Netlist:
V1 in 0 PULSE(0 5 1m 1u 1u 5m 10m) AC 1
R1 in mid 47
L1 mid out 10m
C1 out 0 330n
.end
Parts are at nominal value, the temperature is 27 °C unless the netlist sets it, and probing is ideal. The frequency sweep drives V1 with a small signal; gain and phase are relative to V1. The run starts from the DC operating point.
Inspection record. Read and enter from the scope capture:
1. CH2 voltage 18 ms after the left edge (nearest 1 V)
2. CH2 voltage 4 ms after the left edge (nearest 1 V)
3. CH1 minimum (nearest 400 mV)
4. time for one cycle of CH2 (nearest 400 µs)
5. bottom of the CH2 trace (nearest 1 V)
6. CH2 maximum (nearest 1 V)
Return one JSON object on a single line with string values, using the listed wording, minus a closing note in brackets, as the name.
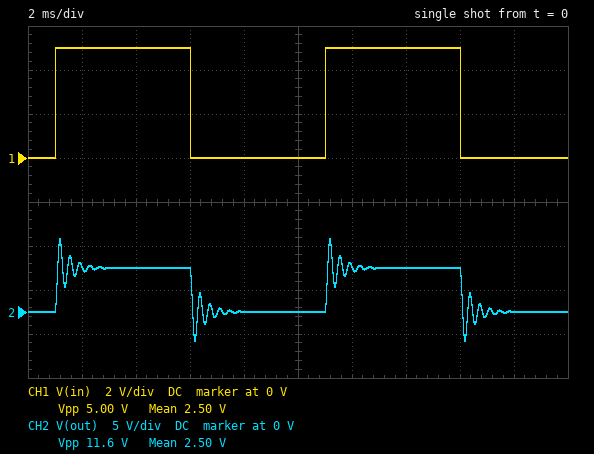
{"CH2 voltage 18 ms after the left edge": "0 V", "CH2 voltage 4 ms after the left edge": "5 V", "CH1 minimum": "0 V", "time for one cycle of CH2": "10.0 ms", "bottom of the CH2 trace": "-3 V", "CH2 maximum": "8 V"}
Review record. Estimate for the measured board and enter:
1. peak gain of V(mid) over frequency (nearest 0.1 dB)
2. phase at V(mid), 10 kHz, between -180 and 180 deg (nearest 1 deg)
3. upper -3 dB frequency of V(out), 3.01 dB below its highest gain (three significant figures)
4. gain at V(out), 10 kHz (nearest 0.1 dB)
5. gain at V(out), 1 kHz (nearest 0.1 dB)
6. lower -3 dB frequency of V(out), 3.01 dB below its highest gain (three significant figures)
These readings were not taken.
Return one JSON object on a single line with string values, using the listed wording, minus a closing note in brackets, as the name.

{"peak gain of V(mid) over frequency": "0 dB", "phase at V(mid), 10 kHz, between -180 and 180 deg": "5 deg", "upper -3 dB frequency of V(out), 3.01 dB below its highest gain": "3.07 kHz", "gain at V(out), 10 kHz": "-21.6 dB", "gain at V(out), 1 kHz": "1.2 dB", "lower -3 dB frequency of V(out), 3.01 dB below its highest gain": "2.31 kHz"}
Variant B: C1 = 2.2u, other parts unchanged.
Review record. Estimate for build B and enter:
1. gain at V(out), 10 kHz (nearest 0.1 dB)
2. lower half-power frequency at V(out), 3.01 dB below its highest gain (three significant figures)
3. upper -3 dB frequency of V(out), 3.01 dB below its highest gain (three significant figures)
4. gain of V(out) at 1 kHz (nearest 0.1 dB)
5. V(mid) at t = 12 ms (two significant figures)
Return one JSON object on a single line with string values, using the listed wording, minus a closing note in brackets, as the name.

{"gain at V(out), 10 kHz": "-38.7 dB", "lower half-power frequency at V(out), 3.01 dB below its highest gain": "345 Hz", "upper -3 dB frequency of V(out), 3.01 dB below its highest gain": "1.27 kHz", "gain of V(out) at 1 kHz": "3.6 dB", "V(mid) at t = 12 ms": "5.0 V"}
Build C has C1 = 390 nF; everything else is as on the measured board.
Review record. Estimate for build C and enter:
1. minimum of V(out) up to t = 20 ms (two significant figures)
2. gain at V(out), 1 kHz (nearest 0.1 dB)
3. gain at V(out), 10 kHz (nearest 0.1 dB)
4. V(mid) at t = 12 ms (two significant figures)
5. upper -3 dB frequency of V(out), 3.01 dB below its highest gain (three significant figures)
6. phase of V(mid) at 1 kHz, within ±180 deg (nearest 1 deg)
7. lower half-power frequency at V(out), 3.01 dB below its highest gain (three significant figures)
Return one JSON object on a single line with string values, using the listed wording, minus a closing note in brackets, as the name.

{"minimum of V(out) up to t = 20 ms": "-3.1 V", "gain at V(out), 1 kHz": "1.4 dB", "gain at V(out), 10 kHz": "-23.2 dB", "V(mid) at t = 12 ms": "5.0 V", "upper -3 dB frequency of V(out), 3.01 dB below its highest gain": "2.85 kHz", "phase of V(mid) at 1 kHz, within ±180 deg": "-8 deg", "lower half-power frequency at V(out), 3.01 dB below its highest gain": "2.08 kHz"}
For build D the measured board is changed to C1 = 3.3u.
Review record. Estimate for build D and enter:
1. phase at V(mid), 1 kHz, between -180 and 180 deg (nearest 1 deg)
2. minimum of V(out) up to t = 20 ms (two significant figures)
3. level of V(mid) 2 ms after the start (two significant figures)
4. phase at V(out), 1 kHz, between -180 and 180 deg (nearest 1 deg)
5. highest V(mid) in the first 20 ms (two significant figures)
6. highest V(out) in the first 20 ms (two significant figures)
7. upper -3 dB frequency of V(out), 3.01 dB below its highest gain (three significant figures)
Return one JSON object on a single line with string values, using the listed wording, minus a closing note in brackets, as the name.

{"phase at V(mid), 1 kHz, between -180 and 180 deg": "73 deg", "minimum of V(out) up to t = 20 ms": "-1.1 V", "level of V(mid) 2 ms after the start": "5.4 V", "phase at V(out), 1 kHz, between -180 and 180 deg": "-107 deg", "highest V(mid) in the first 20 ms": "5.6 V", "highest V(out) in the first 20 ms": "6.1 V", "upper -3 dB frequency of V(out), 3.01 dB below its highest gain": "1.04 kHz"}
